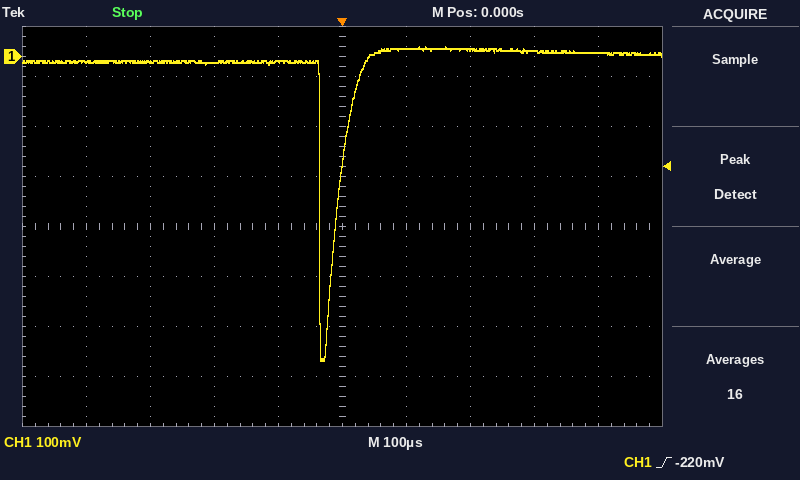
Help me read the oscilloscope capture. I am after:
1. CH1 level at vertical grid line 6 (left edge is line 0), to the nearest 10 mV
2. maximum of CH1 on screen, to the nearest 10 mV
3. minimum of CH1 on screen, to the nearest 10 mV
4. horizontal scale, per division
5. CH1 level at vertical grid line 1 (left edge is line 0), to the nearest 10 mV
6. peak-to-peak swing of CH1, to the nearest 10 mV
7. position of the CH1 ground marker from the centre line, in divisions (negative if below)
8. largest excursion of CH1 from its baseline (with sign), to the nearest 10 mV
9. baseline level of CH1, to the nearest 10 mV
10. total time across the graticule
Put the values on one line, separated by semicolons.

20 mV; 20 mV; -610 mV; 100 µs; -10 mV; 630 mV; +3.4 div; -600 mV; -10 mV; 1 ms
